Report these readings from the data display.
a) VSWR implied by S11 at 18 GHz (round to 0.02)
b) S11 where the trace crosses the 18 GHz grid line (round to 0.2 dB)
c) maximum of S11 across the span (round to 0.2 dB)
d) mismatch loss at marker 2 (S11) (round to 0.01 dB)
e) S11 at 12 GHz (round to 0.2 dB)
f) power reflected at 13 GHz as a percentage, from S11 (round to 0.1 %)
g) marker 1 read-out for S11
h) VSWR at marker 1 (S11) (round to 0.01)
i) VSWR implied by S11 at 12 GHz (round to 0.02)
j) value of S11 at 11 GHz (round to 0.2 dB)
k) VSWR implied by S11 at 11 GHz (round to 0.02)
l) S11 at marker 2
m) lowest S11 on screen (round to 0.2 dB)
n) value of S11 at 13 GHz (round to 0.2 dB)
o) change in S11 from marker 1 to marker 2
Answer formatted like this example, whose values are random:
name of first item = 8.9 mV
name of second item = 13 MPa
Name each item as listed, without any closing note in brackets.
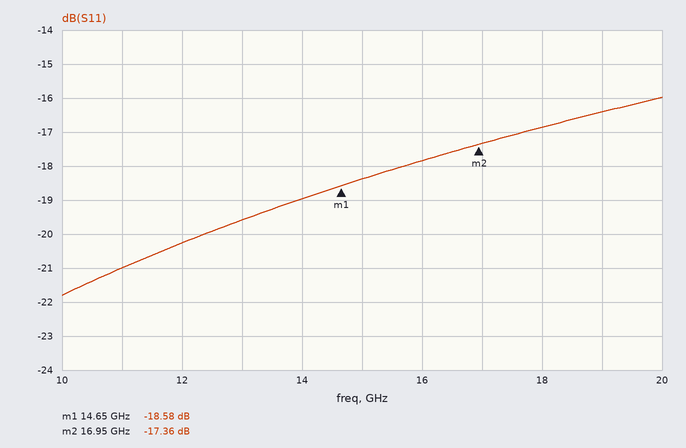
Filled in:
VSWR implied by S11 at 18 GHz = 1.34
S11 where the trace crosses the 18 GHz grid line = -16.8 dB
maximum of S11 across the span = -16.0 dB
mismatch loss at marker 2 (S11) = 0.08 dB
S11 at 12 GHz = -20.2 dB
power reflected at 13 GHz as a percentage, from S11 = 1.1 %
marker 1 read-out for S11 = -18.58 dB
VSWR at marker 1 (S11) = 1.27
VSWR implied by S11 at 12 GHz = 1.22
value of S11 at 11 GHz = -21.0 dB
VSWR implied by S11 at 11 GHz = 1.20
S11 at marker 2 = -17.36 dB
lowest S11 on screen = -21.8 dB
value of S11 at 13 GHz = -19.6 dB
change in S11 from marker 1 to marker 2 = 1.22 dB
